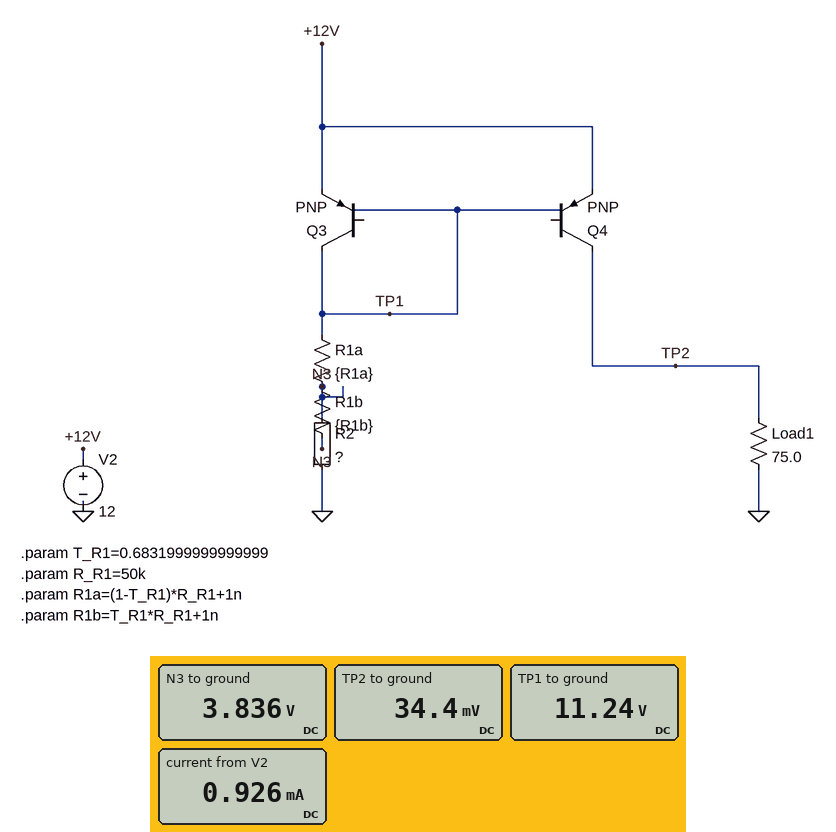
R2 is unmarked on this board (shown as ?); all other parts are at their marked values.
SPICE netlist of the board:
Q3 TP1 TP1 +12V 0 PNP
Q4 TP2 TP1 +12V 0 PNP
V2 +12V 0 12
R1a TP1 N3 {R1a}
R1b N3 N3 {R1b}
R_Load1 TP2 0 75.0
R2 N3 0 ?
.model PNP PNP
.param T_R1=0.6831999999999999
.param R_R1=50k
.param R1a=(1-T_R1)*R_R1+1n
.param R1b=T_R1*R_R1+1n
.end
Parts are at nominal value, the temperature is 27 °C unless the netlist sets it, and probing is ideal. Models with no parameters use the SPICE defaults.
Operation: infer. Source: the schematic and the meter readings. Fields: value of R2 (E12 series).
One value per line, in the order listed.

8.2 kΩ
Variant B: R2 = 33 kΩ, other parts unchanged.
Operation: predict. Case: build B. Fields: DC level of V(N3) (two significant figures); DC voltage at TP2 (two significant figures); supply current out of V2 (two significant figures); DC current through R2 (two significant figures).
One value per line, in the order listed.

7.6 V
17 mV
460 µA
230 µA
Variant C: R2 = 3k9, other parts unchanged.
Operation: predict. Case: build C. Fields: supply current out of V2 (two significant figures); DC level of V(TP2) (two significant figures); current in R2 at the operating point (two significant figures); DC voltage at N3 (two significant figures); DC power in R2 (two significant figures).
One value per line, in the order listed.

1.1 mA
42 mV
570 µA
2.2 V
1.3 mW
